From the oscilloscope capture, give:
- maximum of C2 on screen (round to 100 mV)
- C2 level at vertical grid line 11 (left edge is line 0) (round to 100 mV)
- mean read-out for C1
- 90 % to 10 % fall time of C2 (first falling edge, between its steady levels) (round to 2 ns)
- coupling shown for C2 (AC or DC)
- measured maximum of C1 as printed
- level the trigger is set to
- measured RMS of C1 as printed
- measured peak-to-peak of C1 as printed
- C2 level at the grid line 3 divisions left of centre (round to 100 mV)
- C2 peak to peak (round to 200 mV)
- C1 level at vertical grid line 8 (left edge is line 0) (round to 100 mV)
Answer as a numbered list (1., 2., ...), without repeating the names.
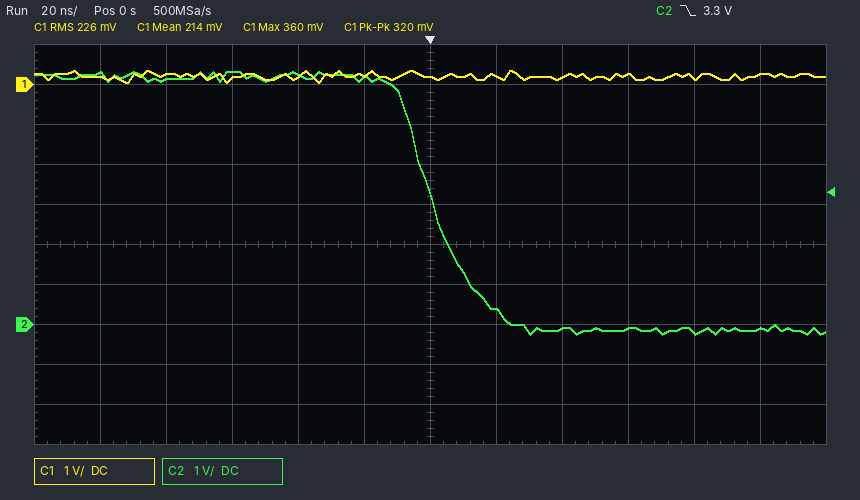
1. 6.3 V
2. -100 mV
3. 214 mV
4. 26 ns
5. DC
6. 360 mV
7. 3.3 V
8. 226 mV
9. 320 mV
10. 6.3 V
11. 6.6 V
12. 200 mV
